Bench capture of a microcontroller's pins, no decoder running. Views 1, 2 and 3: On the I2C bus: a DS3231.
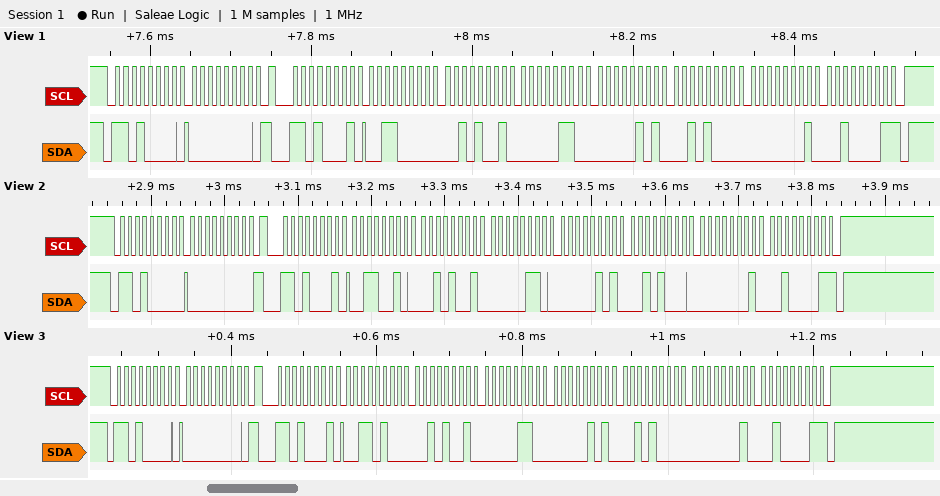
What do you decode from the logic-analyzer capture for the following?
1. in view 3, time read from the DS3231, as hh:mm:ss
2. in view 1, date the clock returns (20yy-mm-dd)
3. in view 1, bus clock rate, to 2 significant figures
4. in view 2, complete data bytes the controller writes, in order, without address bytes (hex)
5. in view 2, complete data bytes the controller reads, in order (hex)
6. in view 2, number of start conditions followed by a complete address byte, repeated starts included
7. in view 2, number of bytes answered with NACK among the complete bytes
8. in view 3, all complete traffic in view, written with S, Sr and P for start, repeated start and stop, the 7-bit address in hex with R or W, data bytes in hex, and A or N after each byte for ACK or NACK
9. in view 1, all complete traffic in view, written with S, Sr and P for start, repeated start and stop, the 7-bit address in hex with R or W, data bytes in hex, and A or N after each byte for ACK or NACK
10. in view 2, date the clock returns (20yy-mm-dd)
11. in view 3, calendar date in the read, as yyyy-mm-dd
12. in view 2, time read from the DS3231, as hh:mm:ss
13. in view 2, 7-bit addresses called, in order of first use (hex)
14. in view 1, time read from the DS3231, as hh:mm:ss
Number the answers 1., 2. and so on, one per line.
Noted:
1. 06:29:34
2. 2021-01-28
3. 100 kHz
4. 00
5. 32 29 06 05 28 01 21
6. 2
7. 1
8. S 68W A 00 A Sr 68R A 34 A 29 A 06 A 05 A 28 A 01 A 21 N P
9. S 68W A 00 A Sr 68R A 30 A 29 A 06 A 05 A 28 A 01 A 21 N P
10. 2021-01-28
11. 2021-01-28
12. 06:29:32
13. 0x68
14. 06:29:30
